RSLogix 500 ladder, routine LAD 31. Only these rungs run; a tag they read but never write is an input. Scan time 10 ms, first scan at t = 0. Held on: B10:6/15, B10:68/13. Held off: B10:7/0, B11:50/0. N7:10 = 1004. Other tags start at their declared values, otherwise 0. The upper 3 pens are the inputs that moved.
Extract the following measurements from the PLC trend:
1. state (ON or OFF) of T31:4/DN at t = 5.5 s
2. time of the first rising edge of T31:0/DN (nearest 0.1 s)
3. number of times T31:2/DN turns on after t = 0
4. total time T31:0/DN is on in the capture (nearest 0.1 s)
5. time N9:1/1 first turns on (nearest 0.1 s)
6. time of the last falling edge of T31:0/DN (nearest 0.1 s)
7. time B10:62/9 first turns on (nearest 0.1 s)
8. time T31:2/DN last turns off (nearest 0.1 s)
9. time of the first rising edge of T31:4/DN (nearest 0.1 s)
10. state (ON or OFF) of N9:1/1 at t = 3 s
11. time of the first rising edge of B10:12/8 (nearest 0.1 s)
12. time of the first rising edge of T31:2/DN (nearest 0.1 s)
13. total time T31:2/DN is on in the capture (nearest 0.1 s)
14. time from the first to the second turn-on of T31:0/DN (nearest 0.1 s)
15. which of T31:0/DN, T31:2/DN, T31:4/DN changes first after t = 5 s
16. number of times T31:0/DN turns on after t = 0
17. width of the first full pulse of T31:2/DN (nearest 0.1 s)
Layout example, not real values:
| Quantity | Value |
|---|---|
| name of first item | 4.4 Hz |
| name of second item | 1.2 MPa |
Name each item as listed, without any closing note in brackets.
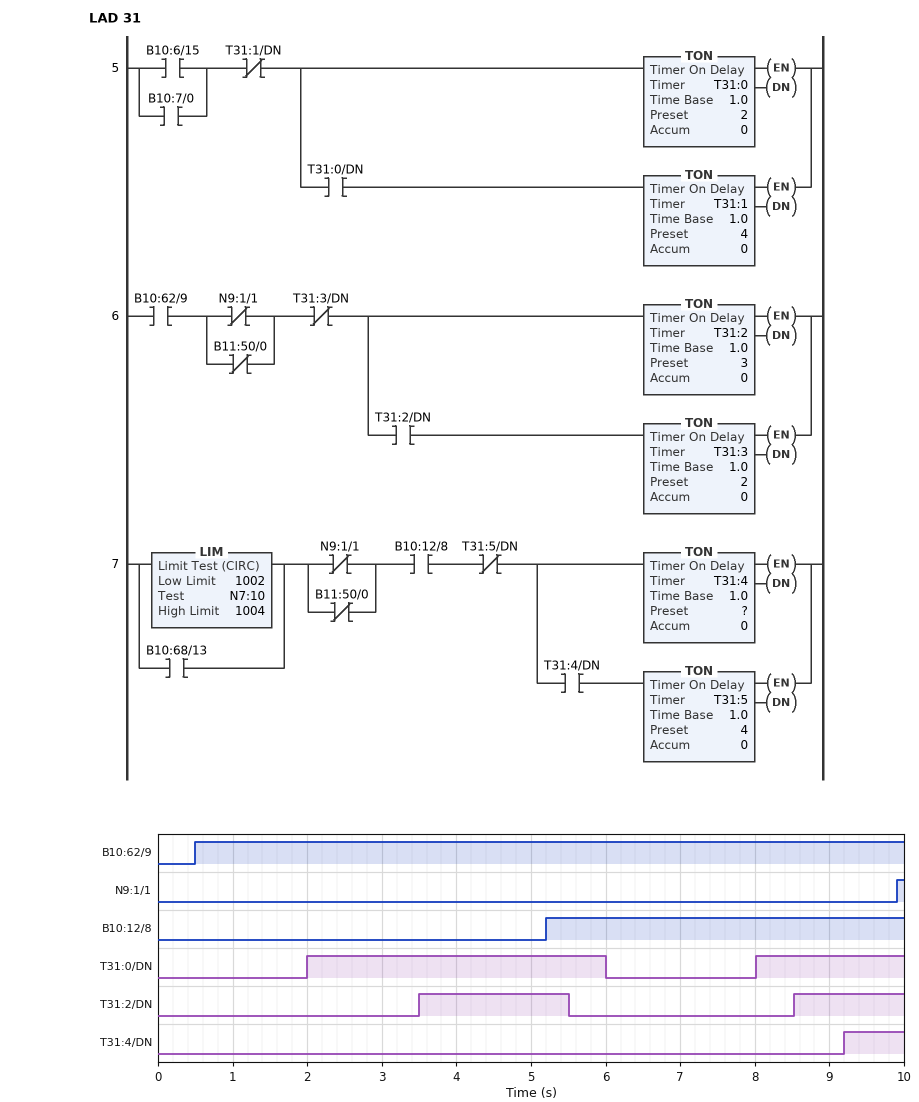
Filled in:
| Quantity | Value |
|---|---|
| state (ON or OFF) of T31:4/DN at t = 5.5 s | OFF |
| time of the first rising edge of T31:0/DN | 2.0 s |
| number of times T31:2/DN turns on after t = 0 | 2 |
| total time T31:0/DN is on in the capture | 6.0 s |
| time N9:1/1 first turns on | 9.9 s |
| time of the last falling edge of T31:0/DN | 6.0 s |
| time B10:62/9 first turns on | 0.5 s |
| time T31:2/DN last turns off | 5.5 s |
| time of the first rising edge of T31:4/DN | 9.2 s |
| state (ON or OFF) of N9:1/1 at t = 3 s | OFF |
| time of the first rising edge of B10:12/8 | 5.2 s |
| time of the first rising edge of T31:2/DN | 3.5 s |
| total time T31:2/DN is on in the capture | 3.5 s |
| time from the first to the second turn-on of T31:0/DN | 6.0 s |
| which of T31:0/DN, T31:2/DN, T31:4/DN changes first after t = 5 s | T31:2/DN |
| number of times T31:0/DN turns on after t = 0 | 2 |
| width of the first full pulse of T31:2/DN | 2.0 s |
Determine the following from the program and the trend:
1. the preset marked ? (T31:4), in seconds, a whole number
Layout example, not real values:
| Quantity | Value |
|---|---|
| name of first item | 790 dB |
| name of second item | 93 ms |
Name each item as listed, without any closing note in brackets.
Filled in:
| Quantity | Value |
|---|---|
| the preset marked ? (T31:4), in seconds, a whole number | 4 s |
